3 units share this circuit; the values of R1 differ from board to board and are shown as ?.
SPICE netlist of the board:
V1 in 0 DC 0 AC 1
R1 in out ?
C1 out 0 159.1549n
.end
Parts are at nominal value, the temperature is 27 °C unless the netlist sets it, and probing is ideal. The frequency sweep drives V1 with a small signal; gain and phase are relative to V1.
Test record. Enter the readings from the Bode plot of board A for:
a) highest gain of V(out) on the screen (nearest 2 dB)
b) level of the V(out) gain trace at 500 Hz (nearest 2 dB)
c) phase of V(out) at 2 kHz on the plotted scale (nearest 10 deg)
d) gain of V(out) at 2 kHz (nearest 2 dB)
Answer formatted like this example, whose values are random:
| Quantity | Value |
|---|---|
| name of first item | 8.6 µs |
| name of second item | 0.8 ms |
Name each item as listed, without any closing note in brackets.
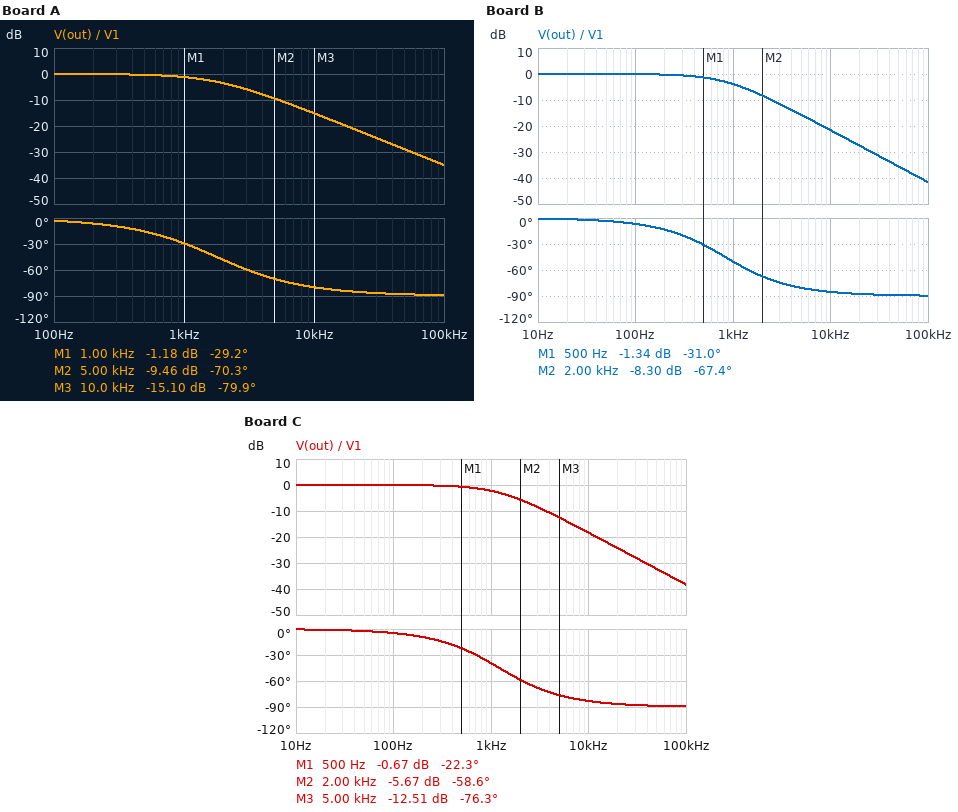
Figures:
| Quantity | Value |
|---|---|
| highest gain of V(out) on the screen | 0 dB |
| level of the V(out) gain trace at 500 Hz | 0 dB |
| phase of V(out) at 2 kHz on the plotted scale | -50 deg |
| gain of V(out) at 2 kHz | -4 dB |
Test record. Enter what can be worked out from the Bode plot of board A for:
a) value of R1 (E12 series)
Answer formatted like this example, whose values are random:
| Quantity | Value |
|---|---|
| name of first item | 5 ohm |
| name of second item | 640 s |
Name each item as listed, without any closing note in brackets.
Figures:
| Quantity | Value |
|---|---|
| value of R1 | 560 Ω |
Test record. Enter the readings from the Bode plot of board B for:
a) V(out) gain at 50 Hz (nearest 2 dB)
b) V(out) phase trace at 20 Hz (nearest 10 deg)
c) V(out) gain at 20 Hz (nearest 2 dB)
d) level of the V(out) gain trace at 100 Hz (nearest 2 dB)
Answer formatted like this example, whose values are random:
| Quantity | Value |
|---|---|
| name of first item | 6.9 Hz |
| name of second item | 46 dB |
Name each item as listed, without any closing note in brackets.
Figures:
| Quantity | Value |
|---|---|
| V(out) gain at 50 Hz | 0 dB |
| V(out) phase trace at 20 Hz | 0 deg |
| V(out) gain at 20 Hz | 0 dB |
| level of the V(out) gain trace at 100 Hz | 0 dB |
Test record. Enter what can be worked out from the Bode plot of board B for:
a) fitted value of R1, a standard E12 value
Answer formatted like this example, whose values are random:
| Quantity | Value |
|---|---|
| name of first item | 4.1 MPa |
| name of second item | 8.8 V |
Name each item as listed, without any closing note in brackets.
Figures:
| Quantity | Value |
|---|---|
| fitted value of R1, a standard E12 value | 1.2 kΩ |
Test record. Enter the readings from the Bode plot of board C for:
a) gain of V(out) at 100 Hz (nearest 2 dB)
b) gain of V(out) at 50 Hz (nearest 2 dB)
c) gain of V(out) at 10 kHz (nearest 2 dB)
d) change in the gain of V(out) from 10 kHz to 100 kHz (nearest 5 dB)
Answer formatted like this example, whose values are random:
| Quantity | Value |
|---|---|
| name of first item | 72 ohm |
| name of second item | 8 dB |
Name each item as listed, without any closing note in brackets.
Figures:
| Quantity | Value |
|---|---|
| gain of V(out) at 100 Hz | 0 dB |
| gain of V(out) at 50 Hz | 0 dB |
| gain of V(out) at 10 kHz | -18 dB |
| change in the gain of V(out) from 10 kHz to 100 kHz | -20 dB |
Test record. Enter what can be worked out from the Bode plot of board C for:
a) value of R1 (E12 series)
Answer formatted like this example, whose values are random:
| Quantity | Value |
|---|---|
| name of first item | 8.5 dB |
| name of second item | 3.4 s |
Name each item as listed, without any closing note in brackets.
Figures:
| Quantity | Value |
|---|---|
| value of R1 | 820 Ω |
